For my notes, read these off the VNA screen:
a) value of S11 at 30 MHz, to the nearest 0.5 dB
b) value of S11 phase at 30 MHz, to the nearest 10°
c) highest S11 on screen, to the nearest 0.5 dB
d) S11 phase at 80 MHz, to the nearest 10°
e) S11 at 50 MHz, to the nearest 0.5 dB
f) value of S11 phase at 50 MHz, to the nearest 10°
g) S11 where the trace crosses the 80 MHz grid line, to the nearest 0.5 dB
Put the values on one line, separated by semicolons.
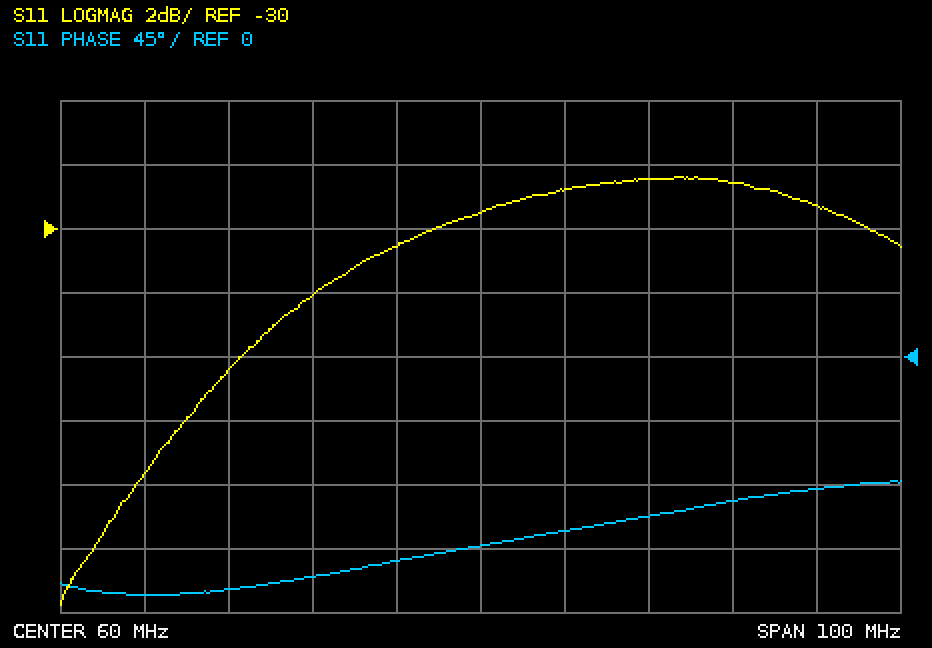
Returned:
-34.5 dB; -160°; -28.5 dB; -110°; -30.5 dB; -140°; -28.5 dB
